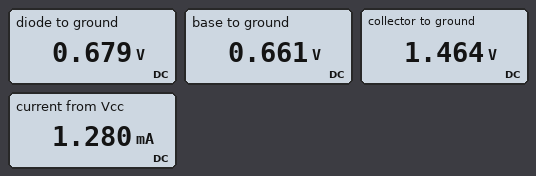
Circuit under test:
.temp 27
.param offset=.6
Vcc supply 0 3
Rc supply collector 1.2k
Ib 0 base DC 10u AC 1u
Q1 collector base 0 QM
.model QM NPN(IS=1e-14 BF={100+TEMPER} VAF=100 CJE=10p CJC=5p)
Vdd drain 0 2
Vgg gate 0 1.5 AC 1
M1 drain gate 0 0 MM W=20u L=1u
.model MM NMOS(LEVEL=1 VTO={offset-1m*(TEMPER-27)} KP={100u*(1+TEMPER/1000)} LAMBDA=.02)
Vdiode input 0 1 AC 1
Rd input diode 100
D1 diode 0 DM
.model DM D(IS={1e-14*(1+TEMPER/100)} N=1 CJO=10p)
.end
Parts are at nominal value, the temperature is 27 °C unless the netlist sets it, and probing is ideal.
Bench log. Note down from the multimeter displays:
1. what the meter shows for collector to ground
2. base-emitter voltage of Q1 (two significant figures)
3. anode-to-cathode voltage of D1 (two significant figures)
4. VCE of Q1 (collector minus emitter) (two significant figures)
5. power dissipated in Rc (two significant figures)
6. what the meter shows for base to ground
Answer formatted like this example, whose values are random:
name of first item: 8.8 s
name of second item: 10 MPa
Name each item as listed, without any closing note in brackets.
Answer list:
what the meter shows for collector to ground: 1.464 V
base-emitter voltage of Q1: 660 mV
anode-to-cathode voltage of D1: 680 mV
VCE of Q1 (collector minus emitter): 1.5 V
power dissipated in Rc: 2.0 mW
what the meter shows for base to ground: 0.661 V
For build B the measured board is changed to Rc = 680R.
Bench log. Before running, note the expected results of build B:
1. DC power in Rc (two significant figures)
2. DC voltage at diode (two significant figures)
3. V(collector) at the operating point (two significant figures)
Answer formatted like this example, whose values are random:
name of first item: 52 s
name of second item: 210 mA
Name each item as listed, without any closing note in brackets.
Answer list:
DC power in Rc: 1.1 mW
DC voltage at diode: 680 mV
V(collector) at the operating point: 2.1 V
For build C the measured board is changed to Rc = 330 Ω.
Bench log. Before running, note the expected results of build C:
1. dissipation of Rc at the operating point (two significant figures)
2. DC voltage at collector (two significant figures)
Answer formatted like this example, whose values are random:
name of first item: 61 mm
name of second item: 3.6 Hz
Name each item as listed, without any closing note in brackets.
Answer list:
dissipation of Rc at the operating point: 550 µW
DC voltage at collector: 2.6 V
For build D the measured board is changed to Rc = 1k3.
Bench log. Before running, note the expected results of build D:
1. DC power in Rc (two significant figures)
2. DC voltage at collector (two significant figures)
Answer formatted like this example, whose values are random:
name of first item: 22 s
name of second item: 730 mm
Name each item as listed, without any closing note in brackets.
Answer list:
DC power in Rc: 2.1 mW
DC voltage at collector: 1.3 V
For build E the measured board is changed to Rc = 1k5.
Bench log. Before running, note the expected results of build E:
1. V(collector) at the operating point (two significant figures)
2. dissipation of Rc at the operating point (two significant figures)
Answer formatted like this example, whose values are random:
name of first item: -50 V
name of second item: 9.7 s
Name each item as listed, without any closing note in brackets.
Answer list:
V(collector) at the operating point: 1.1 V
dissipation of Rc at the operating point: 2.4 mW
